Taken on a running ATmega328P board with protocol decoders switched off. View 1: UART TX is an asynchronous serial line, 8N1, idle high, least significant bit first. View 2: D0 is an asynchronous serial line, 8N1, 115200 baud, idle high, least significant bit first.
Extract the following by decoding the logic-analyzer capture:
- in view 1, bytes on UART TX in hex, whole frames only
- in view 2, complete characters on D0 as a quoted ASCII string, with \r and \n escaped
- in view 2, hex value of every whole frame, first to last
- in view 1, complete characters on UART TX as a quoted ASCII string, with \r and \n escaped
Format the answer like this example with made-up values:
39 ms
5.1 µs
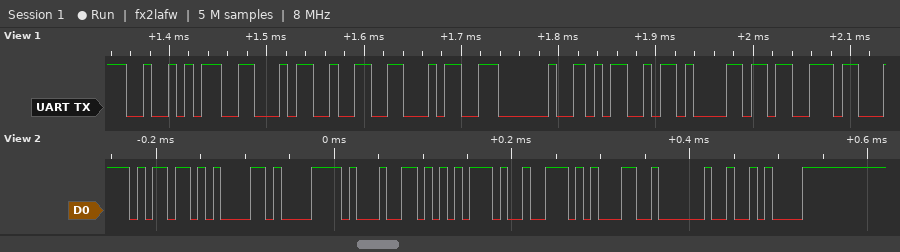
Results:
52 46 32 34 20 4D 61 73
"maxdur1 \n"
6D 61 78 64 75 72 31 20 0A
"RF24 Mas"
